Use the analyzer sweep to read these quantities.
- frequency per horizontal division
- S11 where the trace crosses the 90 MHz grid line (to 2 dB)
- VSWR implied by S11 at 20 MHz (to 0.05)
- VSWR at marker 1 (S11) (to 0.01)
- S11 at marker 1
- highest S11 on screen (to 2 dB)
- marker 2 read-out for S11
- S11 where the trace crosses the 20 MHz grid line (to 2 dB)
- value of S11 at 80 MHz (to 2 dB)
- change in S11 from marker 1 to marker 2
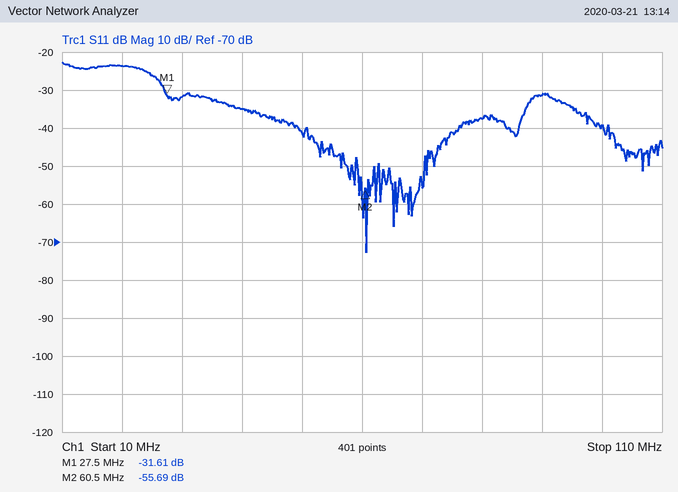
10 MHz
-32 dB
1.15
1.05
-31.61 dB
-22 dB
-55.69 dB
-24 dB
-38 dB
-24.08 dB
